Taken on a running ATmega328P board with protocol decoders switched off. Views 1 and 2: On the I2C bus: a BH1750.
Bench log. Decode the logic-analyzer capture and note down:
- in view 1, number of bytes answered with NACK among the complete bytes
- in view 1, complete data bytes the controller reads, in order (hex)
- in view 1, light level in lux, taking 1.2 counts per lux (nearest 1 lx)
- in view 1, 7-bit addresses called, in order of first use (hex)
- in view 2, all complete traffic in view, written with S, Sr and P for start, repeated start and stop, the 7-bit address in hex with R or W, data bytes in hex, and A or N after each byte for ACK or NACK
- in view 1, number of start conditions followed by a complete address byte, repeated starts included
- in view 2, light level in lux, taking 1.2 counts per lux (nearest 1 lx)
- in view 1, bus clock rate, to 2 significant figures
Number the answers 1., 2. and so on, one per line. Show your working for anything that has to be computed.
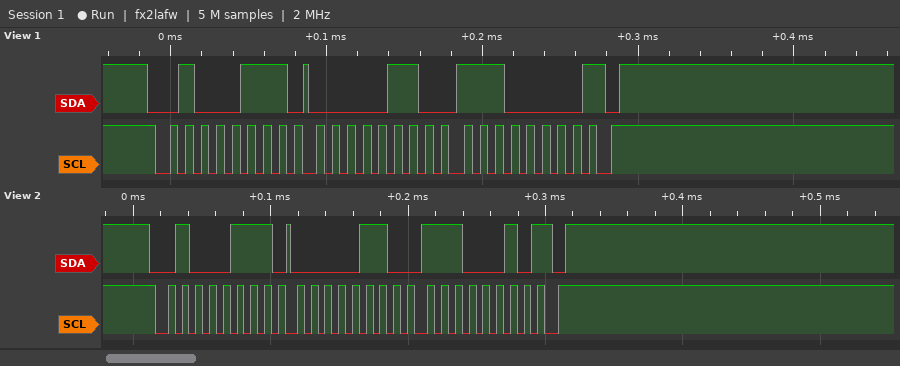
1. 1
2. 06 E0
3. 1760 / 1.2 = 1467 lx
4. 0x23
5. S 23R A 06 A E2 N P
6. 1
7. 1762 / 1.2 = 1468 lx
8. 100 kHz
